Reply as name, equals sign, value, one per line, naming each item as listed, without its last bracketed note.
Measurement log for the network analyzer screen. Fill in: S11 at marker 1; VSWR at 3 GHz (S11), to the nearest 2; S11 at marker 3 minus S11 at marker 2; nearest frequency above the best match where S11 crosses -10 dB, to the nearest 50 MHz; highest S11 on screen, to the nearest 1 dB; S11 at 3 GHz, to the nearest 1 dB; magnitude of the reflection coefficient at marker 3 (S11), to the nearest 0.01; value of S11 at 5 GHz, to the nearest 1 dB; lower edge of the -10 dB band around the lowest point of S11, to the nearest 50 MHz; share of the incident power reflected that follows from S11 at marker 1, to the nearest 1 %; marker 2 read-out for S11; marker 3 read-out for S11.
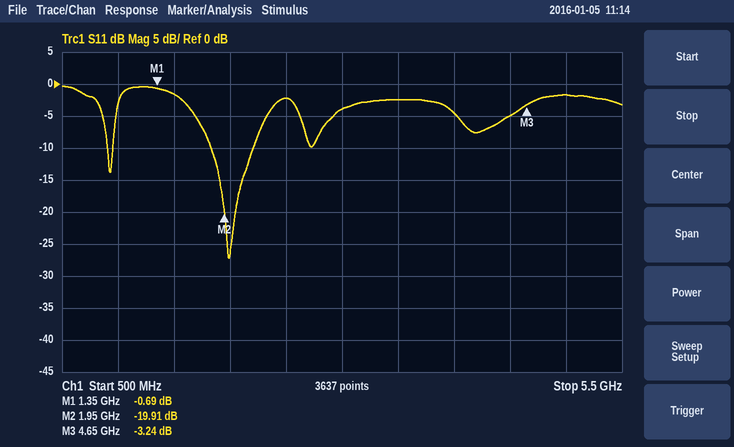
S11 at marker 1 = -0.69 dB
VSWR at 3 GHz (S11), to the nearest 2 = 4
S11 at marker 3 minus S11 at marker 2 = 16.67 dB
nearest frequency above the best match where S11 crosses -10 dB, to the nearest 50 MHz = 2.20 GHz
highest S11 on screen, to the nearest 1 dB = 0 dB
S11 at 3 GHz, to the nearest 1 dB = -4 dB
magnitude of the reflection coefficient at marker 3 (S11), to the nearest 0.01 = 0.69
value of S11 at 5 GHz, to the nearest 1 dB = -2 dB
lower edge of the -10 dB band around the lowest point of S11, to the nearest 50 MHz = 1.85 GHz
share of the incident power reflected that follows from S11 at marker 1, to the nearest 1 % = 85 %
marker 2 read-out for S11 = -19.91 dB
marker 3 read-out for S11 = -3.24 dB
